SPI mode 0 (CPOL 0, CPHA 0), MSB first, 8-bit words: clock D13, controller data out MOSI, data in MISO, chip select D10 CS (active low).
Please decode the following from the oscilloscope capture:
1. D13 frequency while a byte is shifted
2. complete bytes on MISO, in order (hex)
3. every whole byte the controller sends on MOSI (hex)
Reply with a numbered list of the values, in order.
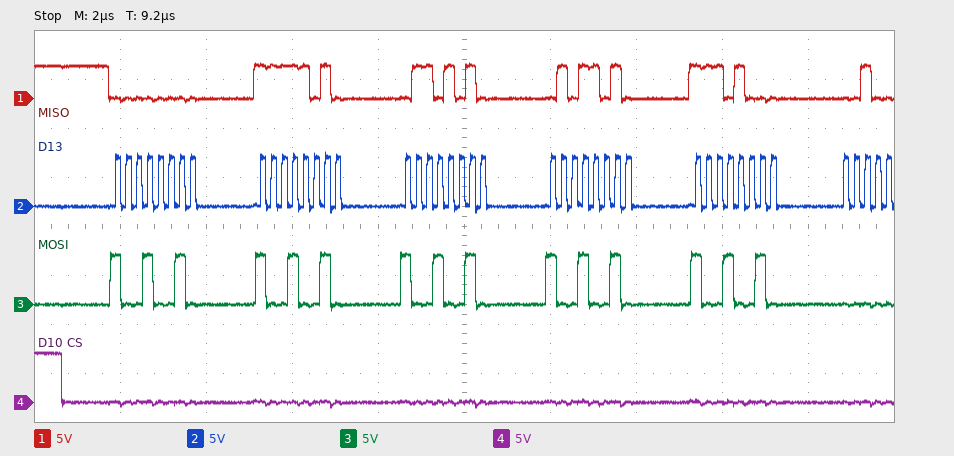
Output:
1. 4 MHz
2. 0x00 0xFA 0x6A 0x5A 0xE8
3. 0x92 0x92 0x92 0x92 0x92
